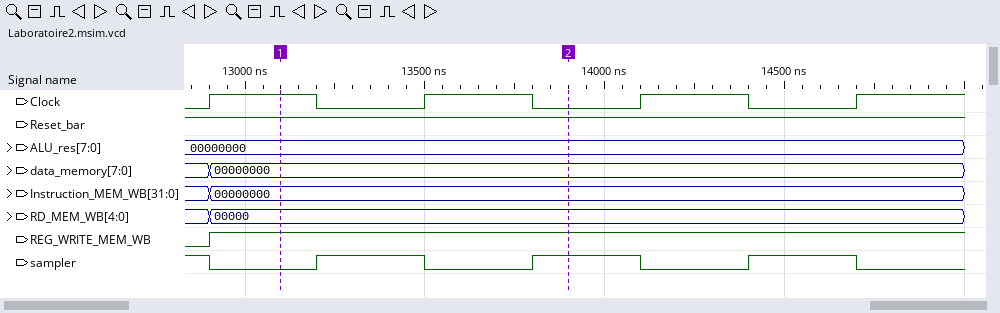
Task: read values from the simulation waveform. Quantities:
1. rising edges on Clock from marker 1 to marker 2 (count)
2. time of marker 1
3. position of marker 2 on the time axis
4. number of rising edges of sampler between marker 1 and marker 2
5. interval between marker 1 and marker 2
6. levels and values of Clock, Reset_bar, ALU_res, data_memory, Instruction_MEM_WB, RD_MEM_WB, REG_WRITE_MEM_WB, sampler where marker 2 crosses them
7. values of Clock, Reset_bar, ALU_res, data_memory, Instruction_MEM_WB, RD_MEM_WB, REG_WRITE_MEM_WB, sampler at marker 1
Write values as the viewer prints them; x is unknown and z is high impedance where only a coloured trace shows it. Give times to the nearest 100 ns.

1
13100 ns
13900 ns
2
800 ns
Clock=0, Reset_bar=1, ALU_res=00000000, data_memory=00000000, Instruction_MEM_WB=00000000, RD_MEM_WB=00000, REG_WRITE_MEM_WB=1, sampler=1
Clock=1, Reset_bar=1, ALU_res=00000000, data_memory=00000000, Instruction_MEM_WB=00000000, RD_MEM_WB=00000, REG_WRITE_MEM_WB=1, sampler=0
